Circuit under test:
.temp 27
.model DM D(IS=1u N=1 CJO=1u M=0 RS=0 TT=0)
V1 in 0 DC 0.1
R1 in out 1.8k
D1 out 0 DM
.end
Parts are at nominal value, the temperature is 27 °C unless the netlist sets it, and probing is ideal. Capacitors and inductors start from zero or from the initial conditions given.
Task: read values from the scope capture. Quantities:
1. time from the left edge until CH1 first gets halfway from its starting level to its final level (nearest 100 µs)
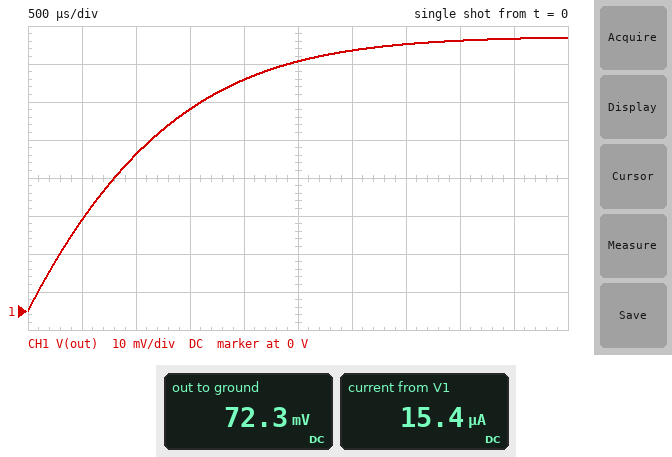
800 µs
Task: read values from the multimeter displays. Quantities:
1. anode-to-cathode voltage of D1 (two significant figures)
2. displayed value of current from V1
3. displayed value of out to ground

72 mV
15.4 µA
72.3 mV
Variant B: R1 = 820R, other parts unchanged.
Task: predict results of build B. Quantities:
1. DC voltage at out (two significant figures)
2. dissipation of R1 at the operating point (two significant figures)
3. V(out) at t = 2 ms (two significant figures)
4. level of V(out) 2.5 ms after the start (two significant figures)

82 mV
410 nW
80 mV
81 mV
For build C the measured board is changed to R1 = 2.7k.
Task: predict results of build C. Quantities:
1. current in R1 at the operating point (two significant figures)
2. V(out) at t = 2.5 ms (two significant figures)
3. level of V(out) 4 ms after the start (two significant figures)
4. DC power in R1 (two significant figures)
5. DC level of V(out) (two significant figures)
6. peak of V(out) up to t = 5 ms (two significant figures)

12 µA
54 mV
63 mV
410 nW
67 mV
65 mV
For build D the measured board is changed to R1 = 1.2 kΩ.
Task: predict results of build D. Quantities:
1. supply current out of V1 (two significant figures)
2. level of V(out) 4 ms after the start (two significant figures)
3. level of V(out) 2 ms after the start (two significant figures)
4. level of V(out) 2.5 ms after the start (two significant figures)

19 µA
77 mV
72 mV
75 mV
